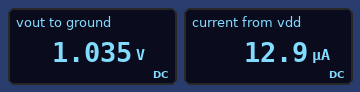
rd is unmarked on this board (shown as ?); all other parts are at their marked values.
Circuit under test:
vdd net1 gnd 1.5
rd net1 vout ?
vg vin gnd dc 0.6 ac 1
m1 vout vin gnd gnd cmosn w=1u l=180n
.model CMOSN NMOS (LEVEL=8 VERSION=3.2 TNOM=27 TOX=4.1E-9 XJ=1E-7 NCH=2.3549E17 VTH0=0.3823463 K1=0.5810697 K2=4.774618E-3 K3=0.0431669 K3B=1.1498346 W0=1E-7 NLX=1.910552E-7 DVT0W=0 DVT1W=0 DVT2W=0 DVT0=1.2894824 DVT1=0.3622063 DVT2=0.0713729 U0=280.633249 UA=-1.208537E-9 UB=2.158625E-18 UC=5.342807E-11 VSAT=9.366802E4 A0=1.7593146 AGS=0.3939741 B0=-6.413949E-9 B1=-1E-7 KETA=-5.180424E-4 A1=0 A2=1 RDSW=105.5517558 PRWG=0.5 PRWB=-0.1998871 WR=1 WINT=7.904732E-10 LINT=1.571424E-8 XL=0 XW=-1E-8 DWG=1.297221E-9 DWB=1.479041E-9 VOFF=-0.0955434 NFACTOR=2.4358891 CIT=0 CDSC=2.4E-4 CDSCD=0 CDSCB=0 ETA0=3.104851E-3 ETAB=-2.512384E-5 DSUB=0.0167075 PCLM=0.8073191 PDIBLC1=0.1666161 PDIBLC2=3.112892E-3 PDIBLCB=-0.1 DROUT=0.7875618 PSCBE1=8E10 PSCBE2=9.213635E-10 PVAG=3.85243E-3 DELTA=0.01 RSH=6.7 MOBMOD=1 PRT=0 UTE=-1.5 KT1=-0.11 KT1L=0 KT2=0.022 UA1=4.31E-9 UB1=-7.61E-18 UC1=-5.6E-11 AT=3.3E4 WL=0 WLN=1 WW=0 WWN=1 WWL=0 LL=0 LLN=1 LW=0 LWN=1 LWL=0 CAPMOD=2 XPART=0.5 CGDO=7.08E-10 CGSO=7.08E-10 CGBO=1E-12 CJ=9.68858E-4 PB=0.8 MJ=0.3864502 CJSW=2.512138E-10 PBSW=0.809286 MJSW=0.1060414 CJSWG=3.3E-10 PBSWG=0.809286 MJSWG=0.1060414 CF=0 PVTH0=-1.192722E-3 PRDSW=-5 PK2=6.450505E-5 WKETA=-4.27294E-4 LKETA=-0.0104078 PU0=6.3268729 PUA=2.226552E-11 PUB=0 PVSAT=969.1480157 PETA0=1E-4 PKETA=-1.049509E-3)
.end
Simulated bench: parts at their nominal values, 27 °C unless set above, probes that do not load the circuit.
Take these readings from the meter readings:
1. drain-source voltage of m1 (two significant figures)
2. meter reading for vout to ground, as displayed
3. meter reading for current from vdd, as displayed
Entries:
1.0 V
1.035 V
12.9 µA
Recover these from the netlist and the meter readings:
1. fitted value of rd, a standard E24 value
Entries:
36 kΩ
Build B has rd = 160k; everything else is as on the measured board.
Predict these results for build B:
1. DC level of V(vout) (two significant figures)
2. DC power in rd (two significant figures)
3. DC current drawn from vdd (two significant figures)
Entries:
150 mV
11 µW
8.4 µA
